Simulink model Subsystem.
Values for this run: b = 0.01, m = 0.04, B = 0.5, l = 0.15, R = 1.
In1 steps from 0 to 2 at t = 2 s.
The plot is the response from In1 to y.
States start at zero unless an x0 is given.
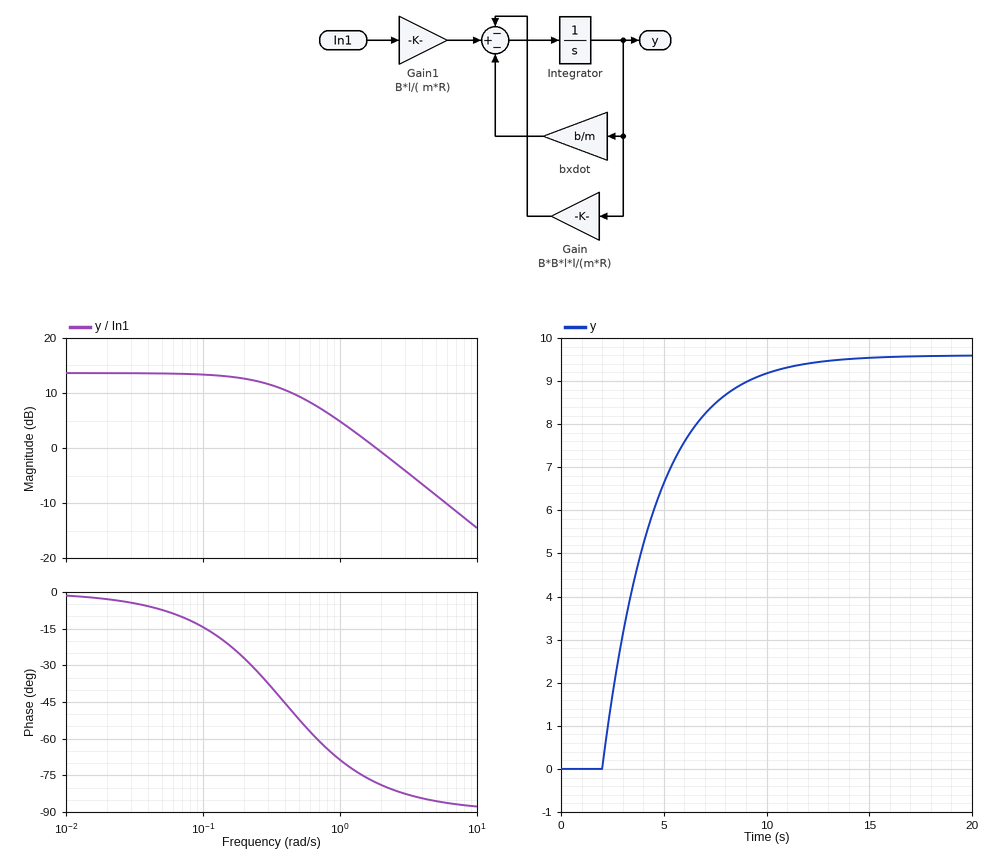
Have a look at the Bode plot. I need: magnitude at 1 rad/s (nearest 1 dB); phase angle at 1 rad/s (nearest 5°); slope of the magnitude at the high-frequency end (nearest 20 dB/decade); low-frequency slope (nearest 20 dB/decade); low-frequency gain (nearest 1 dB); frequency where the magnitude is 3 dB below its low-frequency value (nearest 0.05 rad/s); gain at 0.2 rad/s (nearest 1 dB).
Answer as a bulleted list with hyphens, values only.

- 5 dB
- -70°
- -20 dB/decade
- 0 dB/decade
- 14 dB
- 0.40 rad/s
- 13 dB
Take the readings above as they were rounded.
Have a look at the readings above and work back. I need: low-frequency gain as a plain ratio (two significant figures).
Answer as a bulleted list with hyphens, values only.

- 5.0
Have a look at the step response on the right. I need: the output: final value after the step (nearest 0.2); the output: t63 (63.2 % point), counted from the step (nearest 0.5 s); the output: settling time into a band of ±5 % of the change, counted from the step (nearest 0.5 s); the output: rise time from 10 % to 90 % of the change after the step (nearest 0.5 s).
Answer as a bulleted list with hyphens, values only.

- 9.6
- 2.5 s
- 7.5 s
- 5.5 s
